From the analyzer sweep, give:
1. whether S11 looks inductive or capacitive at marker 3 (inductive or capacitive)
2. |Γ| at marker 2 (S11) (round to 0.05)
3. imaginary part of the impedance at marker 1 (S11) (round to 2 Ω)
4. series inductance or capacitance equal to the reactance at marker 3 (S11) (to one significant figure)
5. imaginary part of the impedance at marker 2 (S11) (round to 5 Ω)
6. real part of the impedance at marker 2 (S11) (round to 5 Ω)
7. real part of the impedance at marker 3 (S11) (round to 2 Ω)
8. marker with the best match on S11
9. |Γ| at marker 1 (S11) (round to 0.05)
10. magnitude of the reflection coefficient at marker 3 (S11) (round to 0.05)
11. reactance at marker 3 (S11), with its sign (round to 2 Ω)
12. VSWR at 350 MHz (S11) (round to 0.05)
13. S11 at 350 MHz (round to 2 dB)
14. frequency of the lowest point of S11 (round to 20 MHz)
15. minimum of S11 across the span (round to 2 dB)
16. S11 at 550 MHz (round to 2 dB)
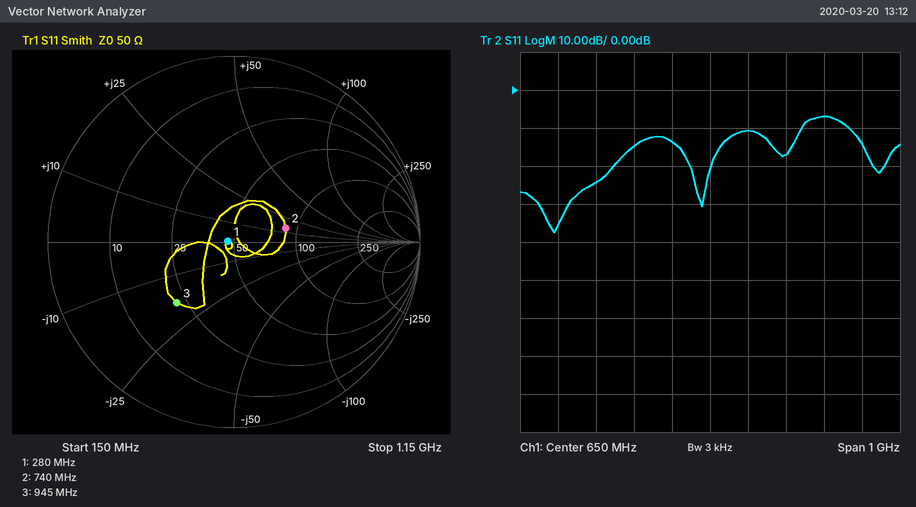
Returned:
capacitive
0.30
0 Ω
9 pF
+15 Ω
85 Ω
22 Ω
marker 1
0.05
0.45
-18 Ω
1.15
-24 dB
240 MHz
-38 dB
-14 dB
